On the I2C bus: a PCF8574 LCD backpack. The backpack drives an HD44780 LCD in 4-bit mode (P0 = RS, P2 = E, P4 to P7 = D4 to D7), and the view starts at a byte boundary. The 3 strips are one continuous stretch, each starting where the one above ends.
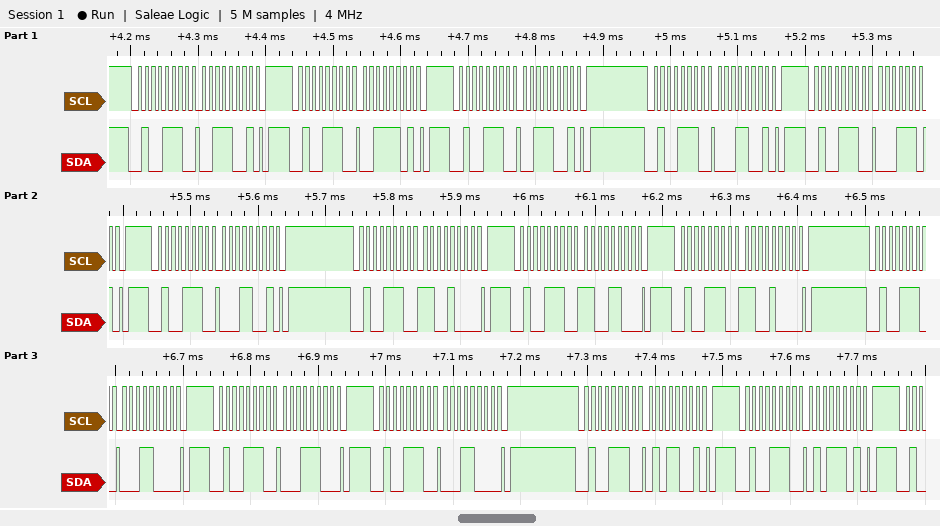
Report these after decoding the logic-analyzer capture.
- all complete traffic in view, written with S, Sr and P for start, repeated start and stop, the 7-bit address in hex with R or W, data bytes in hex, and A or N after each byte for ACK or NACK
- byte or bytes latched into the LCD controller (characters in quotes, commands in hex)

S 27W A 39 A P S 27W A 3D A P S 27W A 39 A P S 27W A 19 A P S 27W A 1D A P S 27W A 19 A P S 27W A C8 A P S 27W A CC A P S 27W A C8 A P S 27W A 18 A P S 27W A 1C A P S 27W A 18 A P S 27W A 59 A P S 27W A 5D A P
'1' 0xC1
